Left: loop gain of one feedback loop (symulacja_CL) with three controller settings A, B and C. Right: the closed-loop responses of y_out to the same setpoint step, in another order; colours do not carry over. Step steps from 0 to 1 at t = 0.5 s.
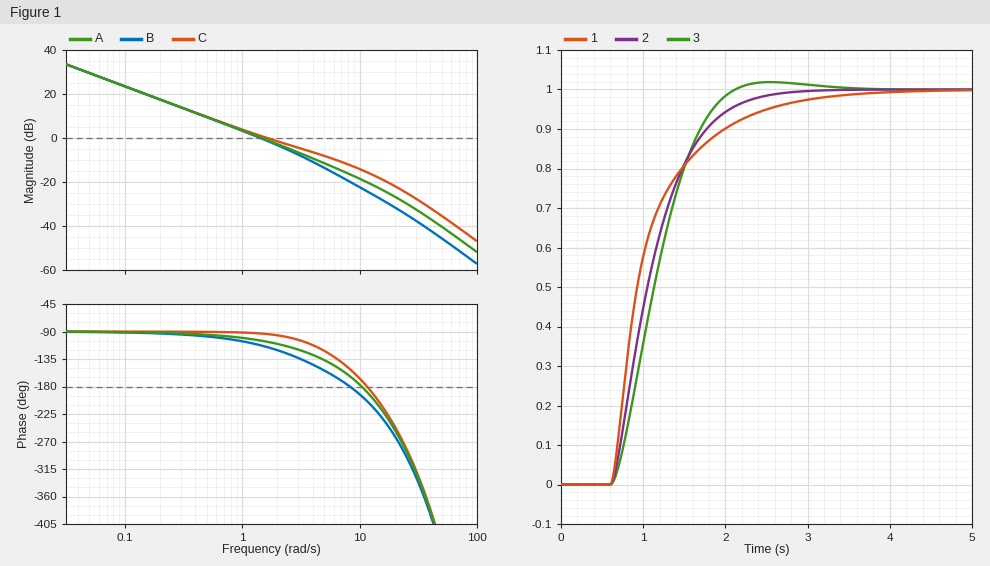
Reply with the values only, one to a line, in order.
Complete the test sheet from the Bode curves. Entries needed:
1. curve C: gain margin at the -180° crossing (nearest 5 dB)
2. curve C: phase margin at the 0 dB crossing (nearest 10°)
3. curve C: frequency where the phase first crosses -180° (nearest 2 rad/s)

15 dB
90°
12 rad/s
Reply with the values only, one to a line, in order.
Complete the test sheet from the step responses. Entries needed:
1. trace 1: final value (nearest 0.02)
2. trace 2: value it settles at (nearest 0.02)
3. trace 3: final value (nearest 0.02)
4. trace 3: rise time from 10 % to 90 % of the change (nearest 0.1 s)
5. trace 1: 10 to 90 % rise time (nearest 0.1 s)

1.00
1.00
1.00
0.9 s
1.3 s
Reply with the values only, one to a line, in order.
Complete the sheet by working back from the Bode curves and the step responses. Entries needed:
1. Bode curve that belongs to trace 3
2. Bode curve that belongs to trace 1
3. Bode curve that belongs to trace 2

B
C
A
